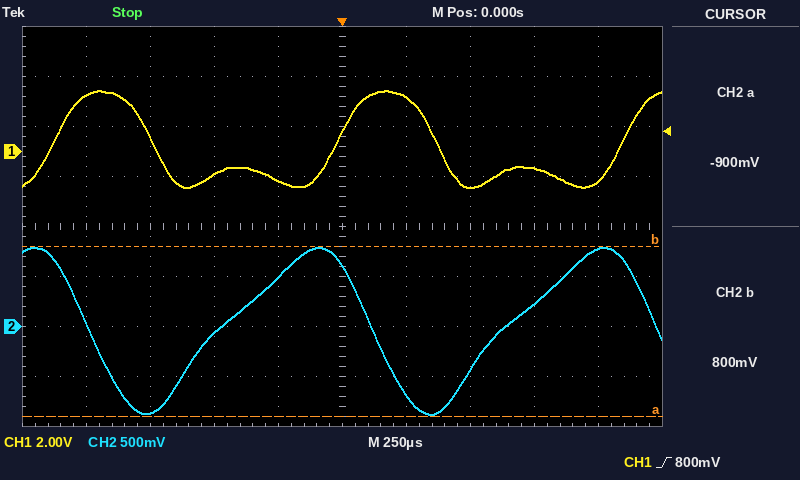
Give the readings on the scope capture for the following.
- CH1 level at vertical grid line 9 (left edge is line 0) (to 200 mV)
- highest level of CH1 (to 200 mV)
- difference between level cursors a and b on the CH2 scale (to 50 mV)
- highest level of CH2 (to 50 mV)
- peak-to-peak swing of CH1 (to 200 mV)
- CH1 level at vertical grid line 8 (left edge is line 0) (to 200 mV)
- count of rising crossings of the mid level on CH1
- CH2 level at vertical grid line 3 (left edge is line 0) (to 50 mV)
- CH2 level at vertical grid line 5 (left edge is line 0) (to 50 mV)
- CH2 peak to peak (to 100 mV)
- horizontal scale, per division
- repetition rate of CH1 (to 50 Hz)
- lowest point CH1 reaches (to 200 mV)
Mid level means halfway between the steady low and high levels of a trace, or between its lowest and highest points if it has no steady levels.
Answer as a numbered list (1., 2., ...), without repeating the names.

1. -1.2 V
2. 2.4 V
3. 1.70 V
4. 800 mV
5. 3.8 V
6. -600 mV
7. 3
8. -50 mV
9. 600 mV
10. 1.70 V
11. 250 µs
12. 900 Hz
13. -1.4 V
